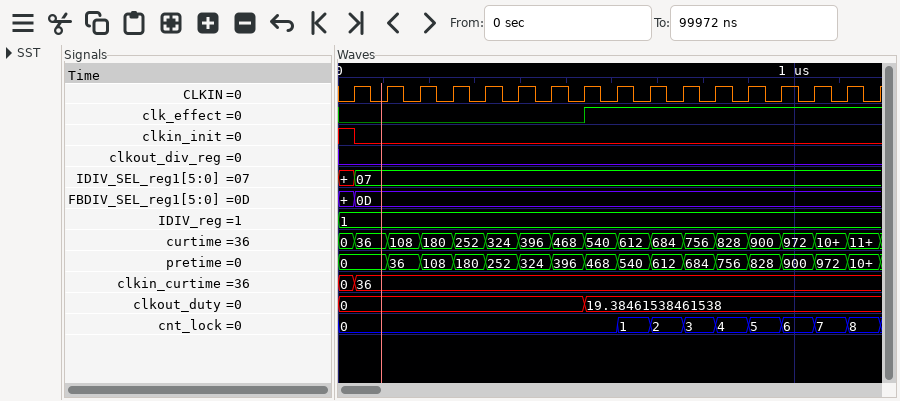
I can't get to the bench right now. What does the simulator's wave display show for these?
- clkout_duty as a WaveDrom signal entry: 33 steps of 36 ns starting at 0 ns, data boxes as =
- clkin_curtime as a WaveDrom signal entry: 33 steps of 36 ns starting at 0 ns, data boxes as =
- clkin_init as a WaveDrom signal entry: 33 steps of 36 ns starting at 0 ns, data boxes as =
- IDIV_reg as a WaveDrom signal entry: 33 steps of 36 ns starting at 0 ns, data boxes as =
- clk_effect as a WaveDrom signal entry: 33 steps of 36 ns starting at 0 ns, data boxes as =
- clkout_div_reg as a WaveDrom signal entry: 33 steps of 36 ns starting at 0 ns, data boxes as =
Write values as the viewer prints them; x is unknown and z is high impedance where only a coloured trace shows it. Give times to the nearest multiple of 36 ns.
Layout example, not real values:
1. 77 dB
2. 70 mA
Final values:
1. {name: 'clkout_duty', wave: '=..............=.................', data: '0 19.38461538461538'}
2. {name: 'clkin_curtime', wave: '==...............................', data: '0 36'}
3. {name: 'clkin_init', wave: '10...............................'}
4. {name: 'IDIV_reg', wave: '=................................', data: '1'}
5. {name: 'clk_effect', wave: '0..............1.................'}
6. {name: 'clkout_div_reg', wave: '0................................'}
